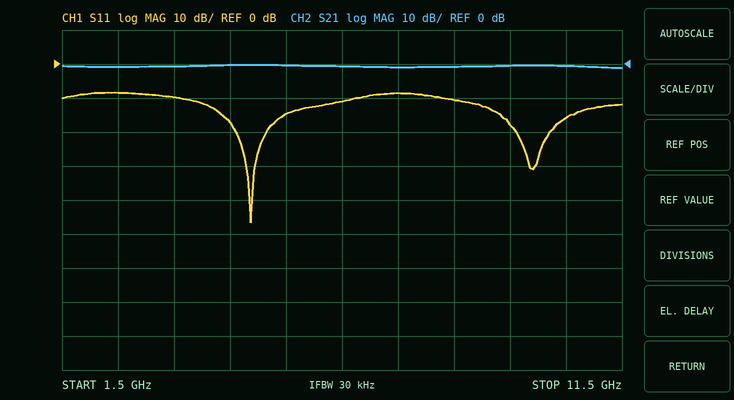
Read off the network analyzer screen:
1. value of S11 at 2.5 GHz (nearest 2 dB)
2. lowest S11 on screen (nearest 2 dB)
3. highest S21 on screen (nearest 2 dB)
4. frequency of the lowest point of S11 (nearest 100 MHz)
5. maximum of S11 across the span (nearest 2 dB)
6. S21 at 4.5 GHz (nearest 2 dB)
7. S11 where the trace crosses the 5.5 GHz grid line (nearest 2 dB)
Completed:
-8 dB
-46 dB
0 dB
4.9 GHz
-8 dB
0 dB
-14 dB
